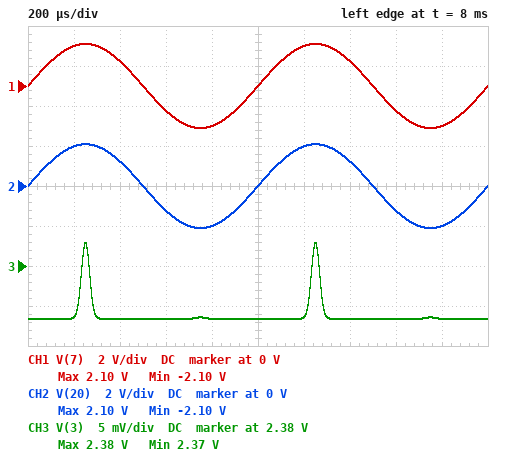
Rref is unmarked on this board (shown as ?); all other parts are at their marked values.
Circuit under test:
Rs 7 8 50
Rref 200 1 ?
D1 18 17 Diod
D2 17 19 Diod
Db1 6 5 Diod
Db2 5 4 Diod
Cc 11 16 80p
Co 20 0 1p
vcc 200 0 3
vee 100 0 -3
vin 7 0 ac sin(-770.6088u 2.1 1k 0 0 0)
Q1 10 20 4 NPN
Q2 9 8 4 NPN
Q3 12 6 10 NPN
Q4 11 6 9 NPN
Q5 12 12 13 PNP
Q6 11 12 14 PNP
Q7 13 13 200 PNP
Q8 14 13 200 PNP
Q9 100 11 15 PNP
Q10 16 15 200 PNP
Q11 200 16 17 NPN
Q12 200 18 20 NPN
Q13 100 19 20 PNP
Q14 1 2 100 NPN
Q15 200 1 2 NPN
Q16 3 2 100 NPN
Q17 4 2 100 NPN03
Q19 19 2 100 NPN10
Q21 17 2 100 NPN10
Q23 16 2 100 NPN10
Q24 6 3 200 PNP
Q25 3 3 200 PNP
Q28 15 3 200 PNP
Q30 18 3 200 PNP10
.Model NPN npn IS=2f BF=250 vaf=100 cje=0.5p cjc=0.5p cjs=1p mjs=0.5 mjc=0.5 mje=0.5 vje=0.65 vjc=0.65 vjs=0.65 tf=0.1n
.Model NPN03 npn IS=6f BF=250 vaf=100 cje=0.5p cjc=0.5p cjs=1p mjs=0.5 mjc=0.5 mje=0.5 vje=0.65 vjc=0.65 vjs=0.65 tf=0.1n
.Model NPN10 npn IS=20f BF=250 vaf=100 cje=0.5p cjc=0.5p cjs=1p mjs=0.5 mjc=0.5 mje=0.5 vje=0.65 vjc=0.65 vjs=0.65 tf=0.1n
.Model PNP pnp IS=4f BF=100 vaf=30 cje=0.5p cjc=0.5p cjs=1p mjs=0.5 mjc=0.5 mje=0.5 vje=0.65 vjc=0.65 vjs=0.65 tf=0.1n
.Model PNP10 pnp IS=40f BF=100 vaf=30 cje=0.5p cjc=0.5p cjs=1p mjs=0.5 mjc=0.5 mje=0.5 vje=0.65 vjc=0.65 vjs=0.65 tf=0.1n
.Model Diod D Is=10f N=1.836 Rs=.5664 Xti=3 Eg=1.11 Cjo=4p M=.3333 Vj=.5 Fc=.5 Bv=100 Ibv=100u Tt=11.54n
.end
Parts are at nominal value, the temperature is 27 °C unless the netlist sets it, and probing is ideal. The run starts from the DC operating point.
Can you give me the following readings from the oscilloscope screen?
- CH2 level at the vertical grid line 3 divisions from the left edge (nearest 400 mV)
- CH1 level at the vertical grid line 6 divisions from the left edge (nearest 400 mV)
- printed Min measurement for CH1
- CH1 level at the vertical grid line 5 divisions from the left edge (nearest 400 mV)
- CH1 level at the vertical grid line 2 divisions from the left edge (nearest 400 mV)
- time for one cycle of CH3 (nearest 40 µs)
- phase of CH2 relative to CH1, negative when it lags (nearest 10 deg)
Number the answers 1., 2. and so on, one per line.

1. -1.2 V
2. 2.0 V
3. -2.10 V
4. 0 V
5. 1.2 V
6. 1.00 ms
7. 0 deg
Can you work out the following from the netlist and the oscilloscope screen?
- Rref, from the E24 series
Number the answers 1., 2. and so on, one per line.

1. 33 kΩ
